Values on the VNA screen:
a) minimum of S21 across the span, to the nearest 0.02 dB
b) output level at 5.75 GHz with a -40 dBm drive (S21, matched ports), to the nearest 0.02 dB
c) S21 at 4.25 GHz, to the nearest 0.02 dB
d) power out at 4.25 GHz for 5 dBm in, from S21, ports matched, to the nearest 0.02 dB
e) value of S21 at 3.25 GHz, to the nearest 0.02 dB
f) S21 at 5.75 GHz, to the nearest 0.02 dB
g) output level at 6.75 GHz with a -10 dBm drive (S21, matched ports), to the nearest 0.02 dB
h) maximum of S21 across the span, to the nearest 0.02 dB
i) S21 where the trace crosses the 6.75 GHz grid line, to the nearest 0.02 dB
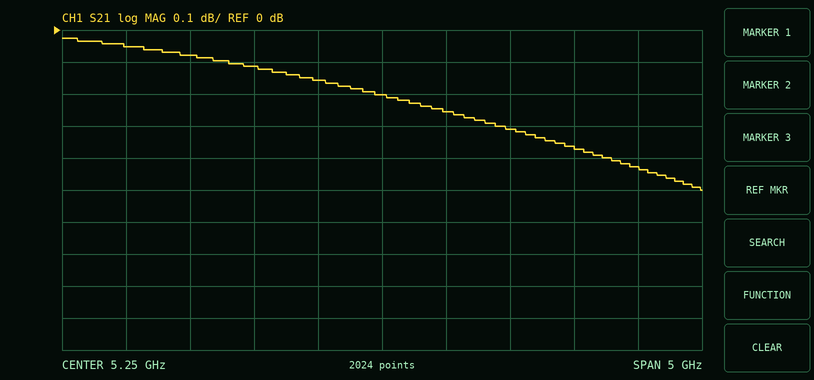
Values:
-0.50 dB
-40.26 dBm
-0.12 dB
4.88 dBm
-0.06 dB
-0.26 dB
-10.36 dBm
-0.02 dB
-0.36 dB
